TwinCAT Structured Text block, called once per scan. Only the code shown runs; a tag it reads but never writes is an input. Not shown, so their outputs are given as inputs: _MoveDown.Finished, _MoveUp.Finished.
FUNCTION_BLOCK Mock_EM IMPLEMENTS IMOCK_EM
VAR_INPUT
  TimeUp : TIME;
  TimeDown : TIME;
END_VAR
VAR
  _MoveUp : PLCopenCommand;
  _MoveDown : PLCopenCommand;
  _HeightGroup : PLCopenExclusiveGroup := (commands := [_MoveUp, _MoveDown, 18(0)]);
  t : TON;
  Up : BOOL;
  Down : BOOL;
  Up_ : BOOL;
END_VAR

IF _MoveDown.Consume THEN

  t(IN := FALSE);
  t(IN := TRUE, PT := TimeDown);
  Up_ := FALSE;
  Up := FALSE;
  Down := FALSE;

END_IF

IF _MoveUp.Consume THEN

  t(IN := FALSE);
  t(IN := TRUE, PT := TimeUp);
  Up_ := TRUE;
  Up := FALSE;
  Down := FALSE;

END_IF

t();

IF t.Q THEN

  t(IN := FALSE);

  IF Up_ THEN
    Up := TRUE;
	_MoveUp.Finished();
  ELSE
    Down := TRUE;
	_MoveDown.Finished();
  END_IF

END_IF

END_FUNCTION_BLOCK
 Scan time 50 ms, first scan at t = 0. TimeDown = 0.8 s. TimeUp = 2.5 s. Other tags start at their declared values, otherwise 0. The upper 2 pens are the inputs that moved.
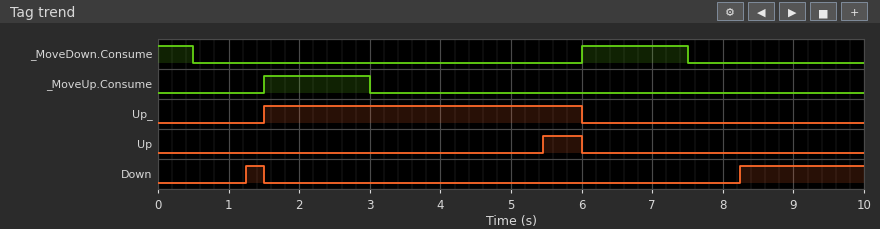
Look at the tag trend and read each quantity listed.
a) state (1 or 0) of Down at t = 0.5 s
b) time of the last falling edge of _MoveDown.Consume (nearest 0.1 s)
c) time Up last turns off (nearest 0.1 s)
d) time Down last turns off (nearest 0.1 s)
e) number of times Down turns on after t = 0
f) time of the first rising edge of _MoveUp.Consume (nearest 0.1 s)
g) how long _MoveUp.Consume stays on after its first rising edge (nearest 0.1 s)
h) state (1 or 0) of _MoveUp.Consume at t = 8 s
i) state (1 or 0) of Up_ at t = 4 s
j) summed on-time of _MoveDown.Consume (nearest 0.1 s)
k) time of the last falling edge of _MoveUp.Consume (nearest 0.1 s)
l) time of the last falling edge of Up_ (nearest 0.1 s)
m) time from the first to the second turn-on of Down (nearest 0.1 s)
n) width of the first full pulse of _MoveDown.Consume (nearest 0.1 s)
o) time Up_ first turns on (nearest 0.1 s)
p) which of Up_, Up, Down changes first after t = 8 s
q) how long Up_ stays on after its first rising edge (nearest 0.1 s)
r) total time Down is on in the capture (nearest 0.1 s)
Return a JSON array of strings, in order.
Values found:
["0", "7.5 s", "6.0 s", "1.5 s", "2", "1.5 s", "1.5 s", "0", "1", "2.0 s", "3.0 s", "6.0 s", "7.0 s", "1.5 s", "1.5 s", "Down", "4.5 s", "2.0 s"]
